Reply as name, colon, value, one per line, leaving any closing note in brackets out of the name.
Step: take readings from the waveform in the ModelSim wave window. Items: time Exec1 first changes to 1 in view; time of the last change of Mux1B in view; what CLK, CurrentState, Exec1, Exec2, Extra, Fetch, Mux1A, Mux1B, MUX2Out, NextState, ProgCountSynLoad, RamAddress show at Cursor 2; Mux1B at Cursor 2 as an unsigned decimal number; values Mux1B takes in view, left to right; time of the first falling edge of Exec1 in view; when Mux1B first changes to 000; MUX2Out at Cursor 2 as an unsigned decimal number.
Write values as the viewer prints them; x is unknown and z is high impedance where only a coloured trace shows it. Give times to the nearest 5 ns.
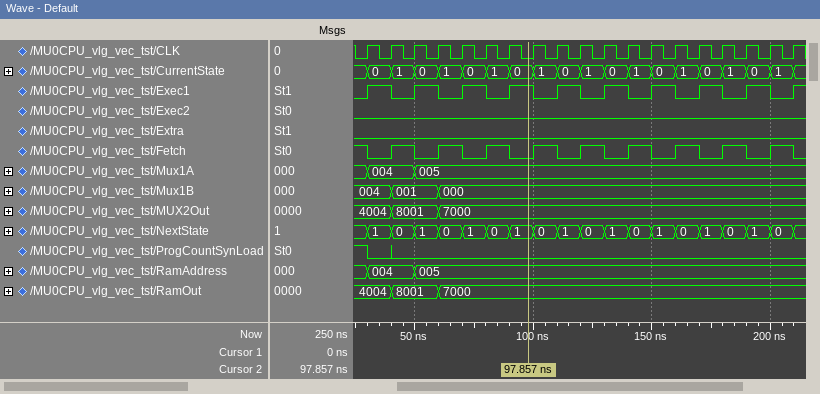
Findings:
time Exec1 first changes to 1 in view: 30 ns
time of the last change of Mux1B in view: 60 ns
what CLK, CurrentState, Exec1, Exec2, Extra, Fetch, Mux1A, Mux1B, MUX2Out, NextState, ProgCountSynLoad, RamAddress show at Cursor 2: CLK=0, CurrentState=0, Exec1=1, Exec2=0, Extra=0, Fetch=0, Mux1A=005, Mux1B=000, MUX2Out=7000, NextState=1, ProgCountSynLoad=0, RamAddress=005
Mux1B at Cursor 2 as an unsigned decimal number: 0
values Mux1B takes in view, left to right: 004, 001, 000
time of the first falling edge of Exec1 in view: 40 ns
when Mux1B first changes to 000: 60 ns
MUX2Out at Cursor 2 as an unsigned decimal number: 28672
